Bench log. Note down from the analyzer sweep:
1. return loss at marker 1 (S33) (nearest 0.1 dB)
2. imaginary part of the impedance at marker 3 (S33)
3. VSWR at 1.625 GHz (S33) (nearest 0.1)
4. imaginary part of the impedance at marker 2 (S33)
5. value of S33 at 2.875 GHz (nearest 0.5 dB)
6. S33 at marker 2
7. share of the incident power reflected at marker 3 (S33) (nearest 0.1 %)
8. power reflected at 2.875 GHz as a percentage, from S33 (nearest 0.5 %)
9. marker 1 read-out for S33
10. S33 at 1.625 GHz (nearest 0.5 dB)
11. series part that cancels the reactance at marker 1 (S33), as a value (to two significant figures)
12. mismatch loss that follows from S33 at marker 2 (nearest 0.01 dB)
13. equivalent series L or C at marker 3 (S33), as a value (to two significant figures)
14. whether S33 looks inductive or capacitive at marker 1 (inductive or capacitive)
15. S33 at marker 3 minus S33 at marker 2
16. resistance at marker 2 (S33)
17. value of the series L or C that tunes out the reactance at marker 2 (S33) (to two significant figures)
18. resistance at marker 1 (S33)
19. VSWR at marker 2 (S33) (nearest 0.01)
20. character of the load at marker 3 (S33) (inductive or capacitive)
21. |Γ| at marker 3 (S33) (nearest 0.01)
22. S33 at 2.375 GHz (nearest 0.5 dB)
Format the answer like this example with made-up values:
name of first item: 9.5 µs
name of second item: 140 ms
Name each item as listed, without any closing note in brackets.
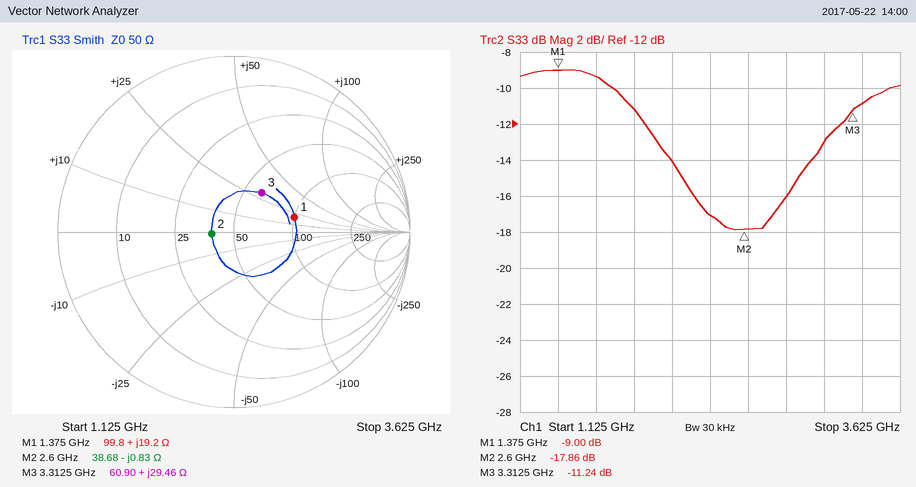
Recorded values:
return loss at marker 1 (S33): 9.0 dB
imaginary part of the impedance at marker 3: +29.46 Ω
VSWR at 1.625 GHz (S33): 2.0
imaginary part of the impedance at marker 2: -0.83 Ω
value of S33 at 2.875 GHz: -16.0 dB
S33 at marker 2: -17.86 dB
share of the incident power reflected at marker 3 (S33): 7.5 %
power reflected at 2.875 GHz as a percentage, from S33: 2.5 %
marker 1 read-out for S33: -9.00 dB
S33 at 1.625 GHz: -9.5 dB
series part that cancels the reactance at marker 1 (S33), as a value: 6.0 pF
mismatch loss that follows from S33 at marker 2: 0.07 dB
equivalent series L or C at marker 3 (S33), as a value: 1.4 nH
whether S33 looks inductive or capacitive at marker 1: inductive
S33 at marker 3 minus S33 at marker 2: 6.62 dB
resistance at marker 2: 38.68 Ω
value of the series L or C that tunes out the reactance at marker 2 (S33): 51 pH
resistance at marker 1: 99.8 Ω
VSWR at marker 2 (S33): 1.29
character of the load at marker 3 (S33): inductive
|Γ| at marker 3 (S33): 0.27
S33 at 2.375 GHz: -17.0 dB
